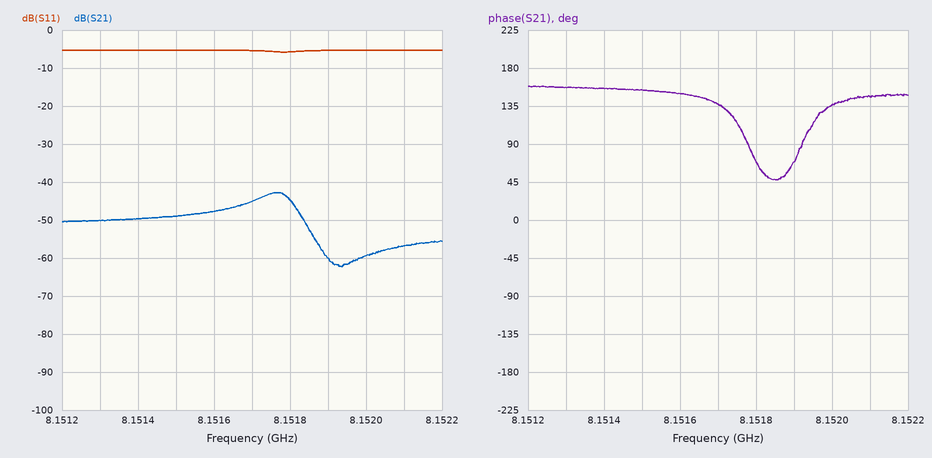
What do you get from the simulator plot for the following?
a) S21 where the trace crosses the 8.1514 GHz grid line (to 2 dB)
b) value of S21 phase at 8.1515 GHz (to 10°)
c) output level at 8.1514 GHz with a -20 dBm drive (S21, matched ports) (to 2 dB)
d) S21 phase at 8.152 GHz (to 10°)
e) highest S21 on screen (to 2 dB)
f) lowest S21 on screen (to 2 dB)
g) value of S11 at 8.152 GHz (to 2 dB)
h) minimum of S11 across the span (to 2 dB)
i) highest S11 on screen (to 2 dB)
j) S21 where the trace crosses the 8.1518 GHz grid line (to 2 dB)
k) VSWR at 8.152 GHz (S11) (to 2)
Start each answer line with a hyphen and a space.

- -50 dB
- 150°
- -70 dBm
- 140°
- -42 dB
- -62 dB
- -6 dB
- -6 dB
- -6 dB
- -44 dB
- 4
